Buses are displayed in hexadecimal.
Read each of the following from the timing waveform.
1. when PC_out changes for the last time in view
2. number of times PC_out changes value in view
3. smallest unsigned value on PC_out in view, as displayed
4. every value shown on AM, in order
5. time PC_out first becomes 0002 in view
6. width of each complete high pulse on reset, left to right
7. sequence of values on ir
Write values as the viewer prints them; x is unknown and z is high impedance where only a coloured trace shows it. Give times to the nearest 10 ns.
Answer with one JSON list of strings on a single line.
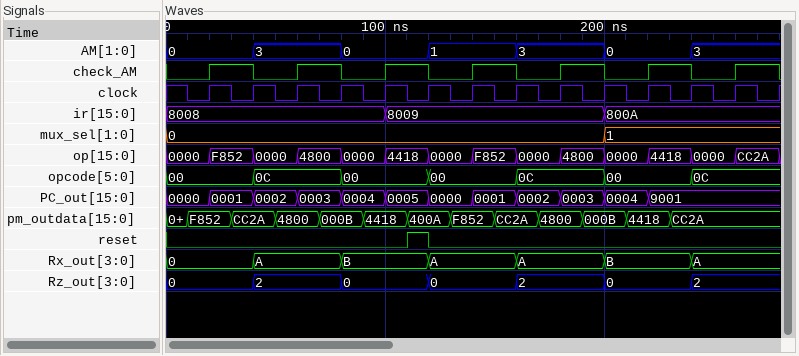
["220 ns", "11", "0000", "0, 3, 0, 1, 3, 0, 3", "40 ns", "10 ns", "8008, 8009, 800A"]
